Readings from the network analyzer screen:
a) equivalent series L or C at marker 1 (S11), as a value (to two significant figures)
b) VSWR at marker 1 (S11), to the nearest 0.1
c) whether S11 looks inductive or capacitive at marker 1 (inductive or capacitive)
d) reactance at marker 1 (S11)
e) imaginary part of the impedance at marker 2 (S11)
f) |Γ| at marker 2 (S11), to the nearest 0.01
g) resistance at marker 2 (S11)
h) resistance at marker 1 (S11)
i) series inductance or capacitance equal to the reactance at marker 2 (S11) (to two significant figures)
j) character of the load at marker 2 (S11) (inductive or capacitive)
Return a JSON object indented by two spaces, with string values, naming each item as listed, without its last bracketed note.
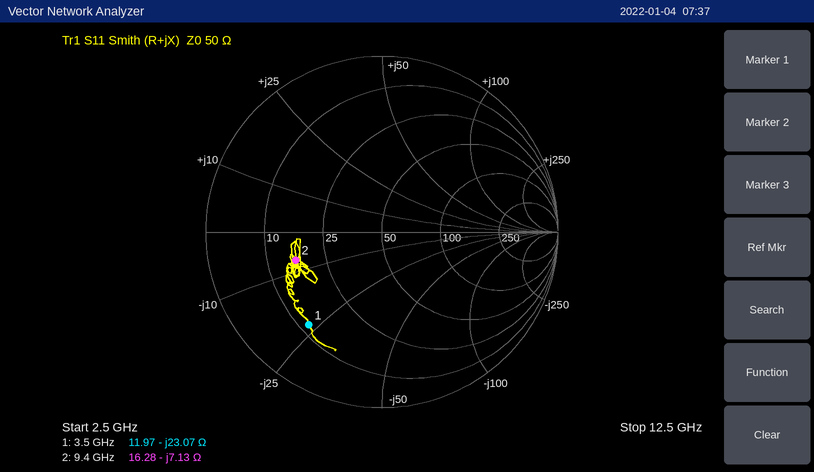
{
  "equivalent series L or C at marker 1 (S11), as a value": "2.0 pF",
  "VSWR at marker 1 (S11), to the nearest 0.1": "5.1",
  "whether S11 looks inductive or capacitive at marker 1": "capacitive",
  "reactance at marker 1": "-23.07 Ω",
  "imaginary part of the impedance at marker 2": "-7.13 Ω",
  "|Γ| at marker 2 (S11), to the nearest 0.01": "0.52",
  "resistance at marker 2": "16.28 Ω",
  "resistance at marker 1": "11.97 Ω",
  "series inductance or capacitance equal to the reactance at marker 2 (S11)": "2.4 pF",
  "character of the load at marker 2 (S11)": "capacitive"
}
